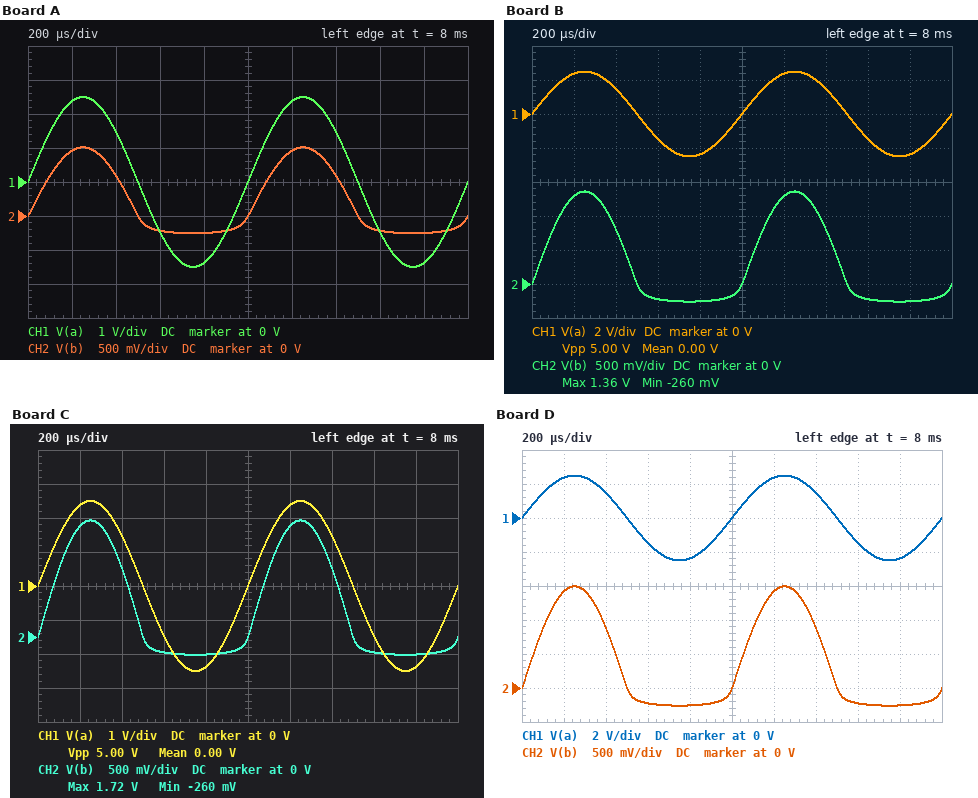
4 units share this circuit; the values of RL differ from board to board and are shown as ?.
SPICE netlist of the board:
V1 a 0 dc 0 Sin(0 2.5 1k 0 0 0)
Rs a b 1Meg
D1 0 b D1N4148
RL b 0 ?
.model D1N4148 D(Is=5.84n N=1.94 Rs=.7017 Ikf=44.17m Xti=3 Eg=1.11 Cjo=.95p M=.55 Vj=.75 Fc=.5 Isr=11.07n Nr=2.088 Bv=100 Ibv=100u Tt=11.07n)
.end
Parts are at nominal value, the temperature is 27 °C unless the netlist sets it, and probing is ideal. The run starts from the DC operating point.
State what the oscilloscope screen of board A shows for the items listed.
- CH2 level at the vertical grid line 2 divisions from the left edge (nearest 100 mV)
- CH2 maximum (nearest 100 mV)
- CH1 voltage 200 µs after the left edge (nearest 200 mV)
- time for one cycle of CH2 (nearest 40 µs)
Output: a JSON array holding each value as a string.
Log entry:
["600 mV", "1.0 V", "2.4 V", "1.00 ms"]
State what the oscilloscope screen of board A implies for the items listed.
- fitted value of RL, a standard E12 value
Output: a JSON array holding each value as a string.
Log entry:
["680 kΩ"]
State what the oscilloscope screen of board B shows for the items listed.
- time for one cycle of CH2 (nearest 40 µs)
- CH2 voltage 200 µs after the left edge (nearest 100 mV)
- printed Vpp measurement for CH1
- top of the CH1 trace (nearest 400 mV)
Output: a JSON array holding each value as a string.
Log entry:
["1.00 ms", "1.3 V", "5.00 V", "2.4 V"]
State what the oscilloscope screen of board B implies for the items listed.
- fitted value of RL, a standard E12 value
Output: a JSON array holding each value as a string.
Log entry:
["1.2 MΩ"]
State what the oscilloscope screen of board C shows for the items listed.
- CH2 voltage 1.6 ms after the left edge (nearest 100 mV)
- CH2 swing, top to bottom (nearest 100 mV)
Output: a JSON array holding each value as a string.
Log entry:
["-200 mV", "2.0 V"]
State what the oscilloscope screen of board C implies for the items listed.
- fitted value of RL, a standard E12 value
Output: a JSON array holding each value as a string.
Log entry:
["2.2 MΩ"]
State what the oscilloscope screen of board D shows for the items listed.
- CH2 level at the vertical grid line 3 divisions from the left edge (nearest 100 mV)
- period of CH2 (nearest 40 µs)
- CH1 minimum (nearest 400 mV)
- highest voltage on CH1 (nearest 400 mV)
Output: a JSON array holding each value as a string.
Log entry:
["-200 mV", "1.00 ms", "-2.4 V", "2.4 V"]
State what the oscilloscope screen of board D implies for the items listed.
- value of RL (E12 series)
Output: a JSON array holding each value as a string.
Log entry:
["1.5 MΩ"]
